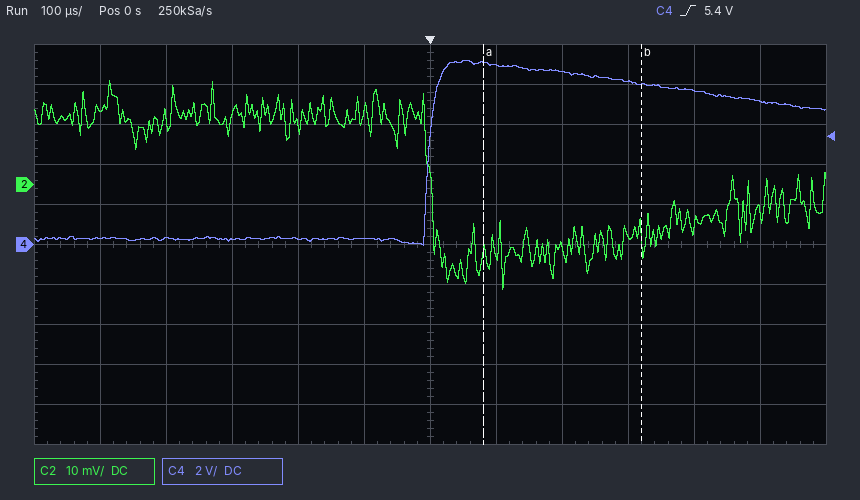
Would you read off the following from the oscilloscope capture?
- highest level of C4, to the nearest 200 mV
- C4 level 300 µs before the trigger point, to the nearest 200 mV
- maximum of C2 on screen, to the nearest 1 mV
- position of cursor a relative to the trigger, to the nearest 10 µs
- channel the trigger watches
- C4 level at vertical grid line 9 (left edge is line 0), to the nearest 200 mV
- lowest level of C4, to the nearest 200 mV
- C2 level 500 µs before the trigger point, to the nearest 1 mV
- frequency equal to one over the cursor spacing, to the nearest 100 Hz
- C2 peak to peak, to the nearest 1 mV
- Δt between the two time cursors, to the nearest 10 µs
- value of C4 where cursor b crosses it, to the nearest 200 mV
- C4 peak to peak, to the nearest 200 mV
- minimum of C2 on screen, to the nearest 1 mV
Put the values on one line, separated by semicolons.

9.2 V; 200 mV; 26 mV; +80 µs; C4; 8.2 V; 0.0 V; 19 mV; 4.2 kHz; 52 mV; 240 µs; 8.0 V; 9.2 V; -26 mV
